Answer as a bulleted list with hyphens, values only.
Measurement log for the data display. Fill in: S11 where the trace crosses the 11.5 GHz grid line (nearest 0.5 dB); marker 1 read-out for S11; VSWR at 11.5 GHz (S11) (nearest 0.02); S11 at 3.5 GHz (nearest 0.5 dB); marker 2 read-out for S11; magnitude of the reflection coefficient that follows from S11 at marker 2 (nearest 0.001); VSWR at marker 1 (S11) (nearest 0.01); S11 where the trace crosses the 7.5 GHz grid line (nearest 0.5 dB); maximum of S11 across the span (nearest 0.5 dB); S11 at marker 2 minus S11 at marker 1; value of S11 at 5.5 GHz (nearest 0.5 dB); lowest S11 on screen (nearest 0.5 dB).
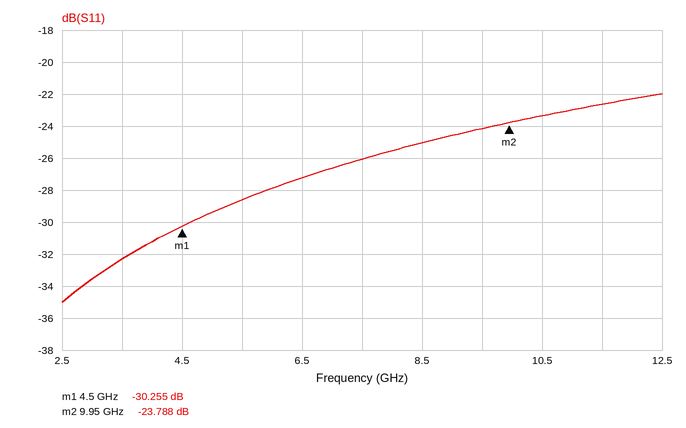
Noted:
- -22.5 dB
- -30.255 dB
- 1.16
- -32.5 dB
- -23.788 dB
- 0.065
- 1.06
- -26.0 dB
- -22.0 dB
- 6.467 dB
- -28.5 dB
- -35.0 dB
